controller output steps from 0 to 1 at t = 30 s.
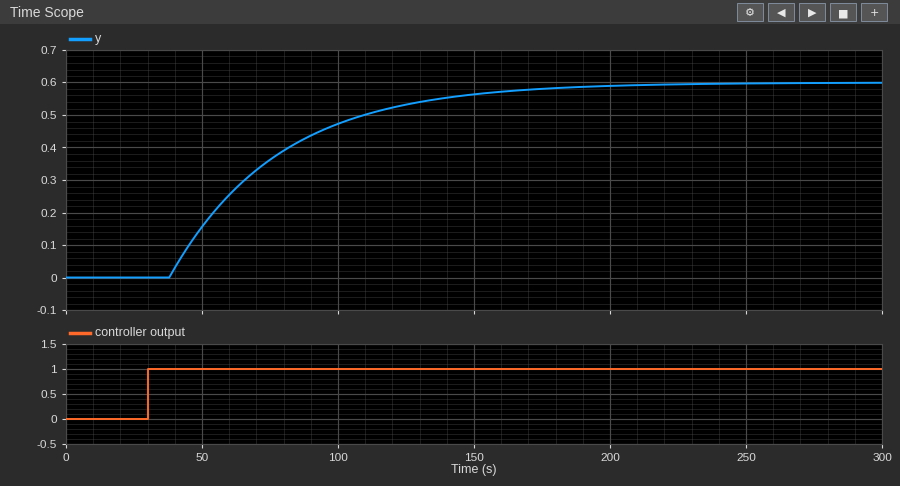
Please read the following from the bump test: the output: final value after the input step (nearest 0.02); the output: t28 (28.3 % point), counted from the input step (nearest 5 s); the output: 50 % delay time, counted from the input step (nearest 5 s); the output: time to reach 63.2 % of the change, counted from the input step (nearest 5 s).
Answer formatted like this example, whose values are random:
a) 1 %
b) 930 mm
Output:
a) 0.60
b) 20 s
c) 35 s
d) 50 s
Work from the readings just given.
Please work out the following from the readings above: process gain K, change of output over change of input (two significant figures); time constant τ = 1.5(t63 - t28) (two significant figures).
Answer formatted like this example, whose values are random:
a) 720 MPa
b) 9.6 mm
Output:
a) 0.60
b) 45 s
